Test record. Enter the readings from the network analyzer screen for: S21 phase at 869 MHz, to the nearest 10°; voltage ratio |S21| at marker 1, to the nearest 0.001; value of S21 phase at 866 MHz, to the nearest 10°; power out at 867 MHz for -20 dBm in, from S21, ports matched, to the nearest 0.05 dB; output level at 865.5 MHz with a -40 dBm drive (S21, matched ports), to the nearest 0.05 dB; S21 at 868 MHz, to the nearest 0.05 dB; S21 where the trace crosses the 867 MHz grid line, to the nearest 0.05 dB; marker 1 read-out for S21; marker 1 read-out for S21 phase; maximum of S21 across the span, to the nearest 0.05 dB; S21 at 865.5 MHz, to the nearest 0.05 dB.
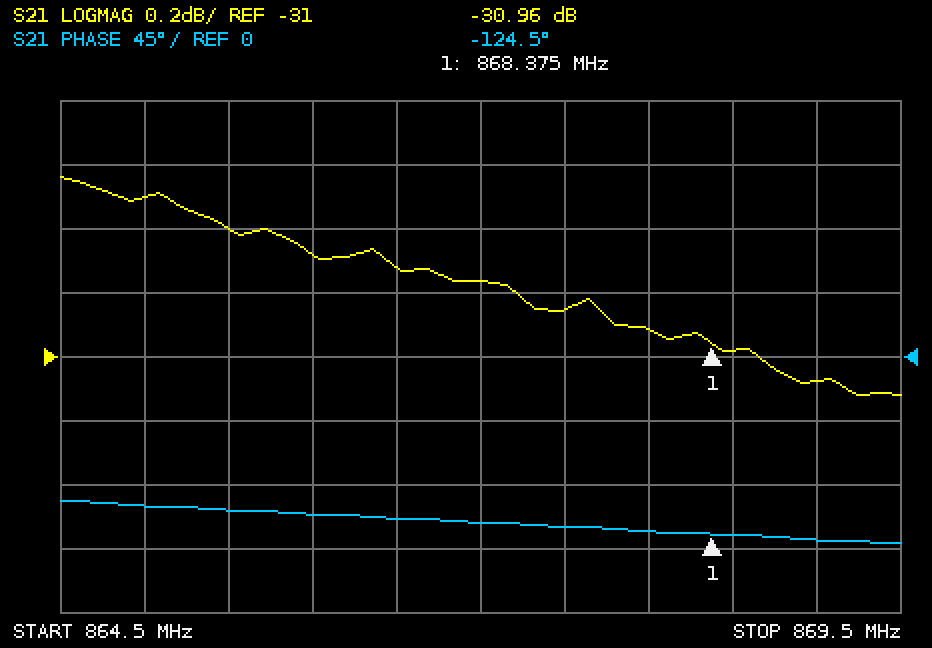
-130°
0.028
-110°
-50.75 dBm
-70.60 dBm
-30.90 dB
-30.75 dB
-30.96 dB
-124.5°
-30.45 dB
-30.60 dB
